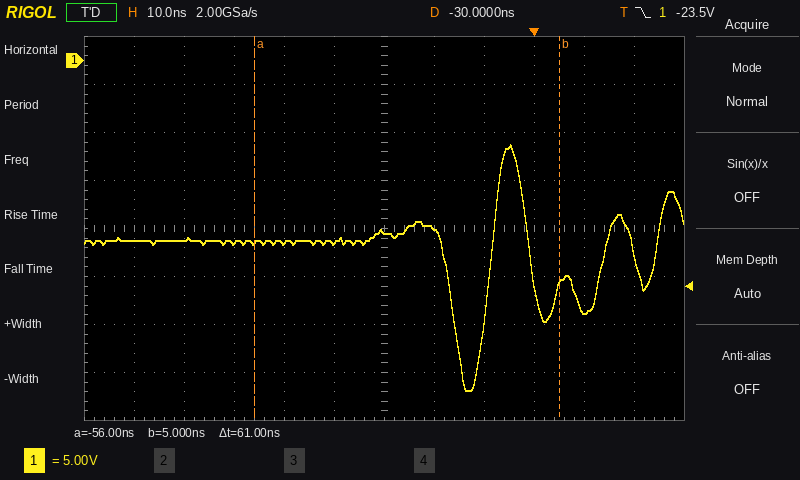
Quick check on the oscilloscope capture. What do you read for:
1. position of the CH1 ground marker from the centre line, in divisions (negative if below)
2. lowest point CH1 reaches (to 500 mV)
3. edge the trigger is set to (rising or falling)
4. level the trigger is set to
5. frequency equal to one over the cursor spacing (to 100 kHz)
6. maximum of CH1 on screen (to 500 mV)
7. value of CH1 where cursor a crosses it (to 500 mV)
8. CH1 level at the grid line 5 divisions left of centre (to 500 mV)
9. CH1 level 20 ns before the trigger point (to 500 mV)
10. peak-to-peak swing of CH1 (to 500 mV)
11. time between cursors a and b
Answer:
+3.5 div
-34.5 V
falling
-23.5 V
16.4 MHz
-9.0 V
-19.0 V
-19.0 V
-17.5 V
25.5 V
61 ns
